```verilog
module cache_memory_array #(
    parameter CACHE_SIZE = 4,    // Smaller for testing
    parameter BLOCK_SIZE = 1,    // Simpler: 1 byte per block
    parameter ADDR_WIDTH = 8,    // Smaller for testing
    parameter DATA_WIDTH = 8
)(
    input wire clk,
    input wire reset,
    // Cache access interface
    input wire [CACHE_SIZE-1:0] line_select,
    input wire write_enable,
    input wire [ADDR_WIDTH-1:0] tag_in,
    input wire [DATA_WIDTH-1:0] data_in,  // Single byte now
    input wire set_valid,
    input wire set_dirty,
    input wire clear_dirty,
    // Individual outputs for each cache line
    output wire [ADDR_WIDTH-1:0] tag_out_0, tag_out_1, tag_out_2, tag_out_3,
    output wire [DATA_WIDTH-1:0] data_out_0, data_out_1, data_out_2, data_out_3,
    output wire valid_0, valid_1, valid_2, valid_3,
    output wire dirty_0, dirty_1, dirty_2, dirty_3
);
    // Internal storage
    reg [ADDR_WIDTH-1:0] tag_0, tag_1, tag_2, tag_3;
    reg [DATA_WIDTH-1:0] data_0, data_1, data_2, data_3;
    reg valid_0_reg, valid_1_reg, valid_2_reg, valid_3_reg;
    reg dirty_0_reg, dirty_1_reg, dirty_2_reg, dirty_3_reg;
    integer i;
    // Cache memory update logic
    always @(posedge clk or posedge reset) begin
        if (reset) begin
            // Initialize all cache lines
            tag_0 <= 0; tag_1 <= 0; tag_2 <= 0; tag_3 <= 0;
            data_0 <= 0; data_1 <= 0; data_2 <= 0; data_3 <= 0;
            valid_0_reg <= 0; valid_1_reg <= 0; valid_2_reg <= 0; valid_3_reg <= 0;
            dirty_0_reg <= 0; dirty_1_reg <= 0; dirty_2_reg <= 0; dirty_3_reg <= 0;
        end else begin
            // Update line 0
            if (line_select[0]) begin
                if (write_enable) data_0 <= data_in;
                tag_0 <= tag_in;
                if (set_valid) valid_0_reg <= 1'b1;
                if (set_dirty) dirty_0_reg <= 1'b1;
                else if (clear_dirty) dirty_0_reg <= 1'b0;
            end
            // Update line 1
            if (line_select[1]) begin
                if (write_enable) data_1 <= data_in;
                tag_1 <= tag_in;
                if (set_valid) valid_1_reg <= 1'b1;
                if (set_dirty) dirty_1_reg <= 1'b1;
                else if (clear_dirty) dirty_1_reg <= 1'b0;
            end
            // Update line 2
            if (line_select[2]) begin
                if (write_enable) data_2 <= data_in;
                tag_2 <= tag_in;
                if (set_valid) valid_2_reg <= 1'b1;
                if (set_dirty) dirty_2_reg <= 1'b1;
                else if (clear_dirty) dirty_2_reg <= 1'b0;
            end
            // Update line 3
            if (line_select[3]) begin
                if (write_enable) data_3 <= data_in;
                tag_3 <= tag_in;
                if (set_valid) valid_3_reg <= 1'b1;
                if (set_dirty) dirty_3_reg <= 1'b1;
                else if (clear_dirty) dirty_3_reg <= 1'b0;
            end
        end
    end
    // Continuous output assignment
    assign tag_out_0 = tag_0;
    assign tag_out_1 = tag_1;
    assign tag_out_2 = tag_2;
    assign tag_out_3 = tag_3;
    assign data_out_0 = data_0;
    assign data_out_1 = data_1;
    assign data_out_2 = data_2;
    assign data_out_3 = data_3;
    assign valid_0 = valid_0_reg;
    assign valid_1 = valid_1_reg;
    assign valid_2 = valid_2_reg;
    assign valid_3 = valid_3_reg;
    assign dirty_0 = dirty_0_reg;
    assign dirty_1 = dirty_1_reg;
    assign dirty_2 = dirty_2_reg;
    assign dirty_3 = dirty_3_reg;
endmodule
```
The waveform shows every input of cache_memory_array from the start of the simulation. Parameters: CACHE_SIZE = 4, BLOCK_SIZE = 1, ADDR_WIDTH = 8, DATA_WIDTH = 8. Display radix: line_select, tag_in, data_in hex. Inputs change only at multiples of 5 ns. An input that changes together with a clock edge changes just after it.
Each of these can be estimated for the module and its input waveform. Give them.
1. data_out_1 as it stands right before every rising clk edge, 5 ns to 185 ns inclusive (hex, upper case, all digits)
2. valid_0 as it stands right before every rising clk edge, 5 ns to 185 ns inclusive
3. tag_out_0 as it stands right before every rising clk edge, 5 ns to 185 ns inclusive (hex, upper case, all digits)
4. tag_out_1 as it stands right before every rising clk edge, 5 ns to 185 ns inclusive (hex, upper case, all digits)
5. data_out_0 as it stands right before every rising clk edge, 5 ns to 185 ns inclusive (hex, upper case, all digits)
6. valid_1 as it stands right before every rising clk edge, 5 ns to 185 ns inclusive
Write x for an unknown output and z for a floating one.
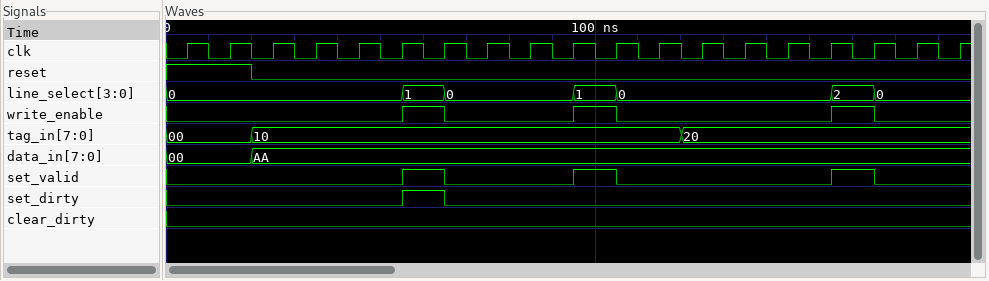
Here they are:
00, 00, 00, 00, 00, 00, 00, 00, 00, 00, 00, 00, 00, 00, 00, 00, 00, AA, AA
0 0 0 0 0 0 0 1 1 1 1 1 1 1 1 1 1 1 1
00, 00, 00, 00, 00, 00, 00, 10, 10, 10, 10, 10, 10, 10, 10, 10, 10, 10, 10
00, 00, 00, 00, 00, 00, 00, 00, 00, 00, 00, 00, 00, 00, 00, 00, 00, 20, 20
00, 00, 00, 00, 00, 00, 00, AA, AA, AA, AA, AA, AA, AA, AA, AA, AA, AA, AA
0 0 0 0 0 0 0 0 0 0 0 0 0 0 0 0 0 1 1
